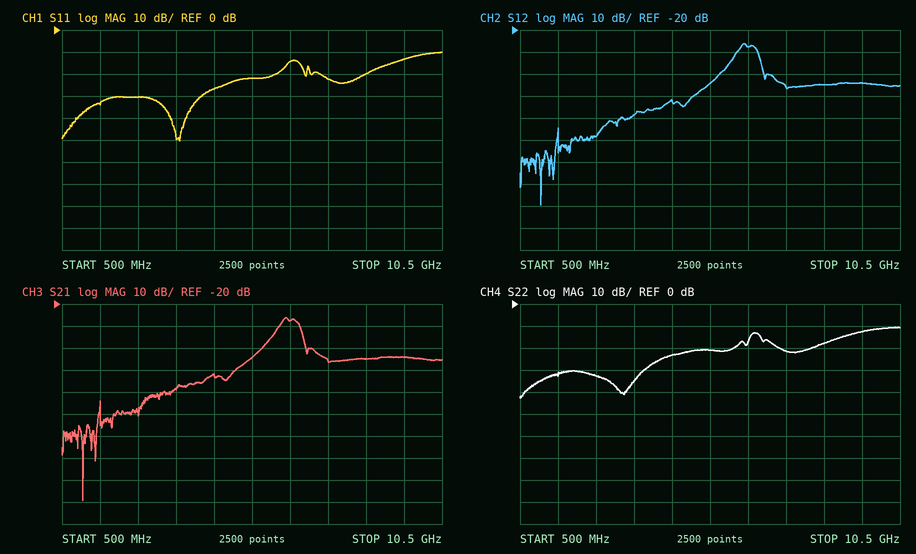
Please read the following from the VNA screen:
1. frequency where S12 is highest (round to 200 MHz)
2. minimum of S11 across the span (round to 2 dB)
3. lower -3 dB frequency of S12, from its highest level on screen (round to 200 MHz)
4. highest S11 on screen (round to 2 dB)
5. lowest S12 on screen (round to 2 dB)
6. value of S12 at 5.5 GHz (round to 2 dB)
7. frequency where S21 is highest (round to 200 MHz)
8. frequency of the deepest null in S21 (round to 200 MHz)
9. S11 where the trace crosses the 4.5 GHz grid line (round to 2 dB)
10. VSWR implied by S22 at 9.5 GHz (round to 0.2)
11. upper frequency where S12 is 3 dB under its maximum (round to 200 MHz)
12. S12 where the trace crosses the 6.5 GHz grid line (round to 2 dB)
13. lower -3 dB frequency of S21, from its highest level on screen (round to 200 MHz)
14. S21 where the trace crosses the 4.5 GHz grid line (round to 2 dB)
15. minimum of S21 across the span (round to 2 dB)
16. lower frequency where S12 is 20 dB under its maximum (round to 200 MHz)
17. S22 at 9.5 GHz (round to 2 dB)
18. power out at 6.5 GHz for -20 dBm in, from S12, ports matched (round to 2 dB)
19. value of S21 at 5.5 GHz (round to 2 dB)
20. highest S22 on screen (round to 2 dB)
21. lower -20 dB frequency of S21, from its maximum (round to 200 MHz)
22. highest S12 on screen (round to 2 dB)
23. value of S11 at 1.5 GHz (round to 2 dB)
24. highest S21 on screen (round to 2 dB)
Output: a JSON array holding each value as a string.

["6.4 GHz", "-50 dB", "6.2 GHz", "-10 dB", "-100 dB", "-44 dB", "6.4 GHz", "1.0 GHz", "-26 dB", "1.6", "6.8 GHz", "-28 dB", "6.2 GHz", "-52 dB", "-110 dB", "5.4 GHz", "-12 dB", "-48 dBm", "-44 dB", "-10 dB", "5.4 GHz", "-26 dB", "-34 dB", "-26 dB"]
